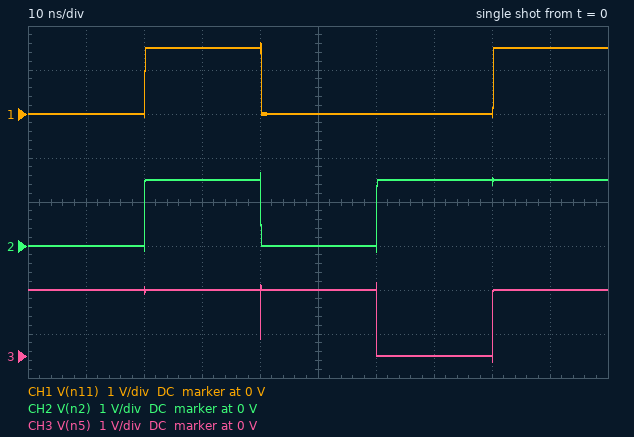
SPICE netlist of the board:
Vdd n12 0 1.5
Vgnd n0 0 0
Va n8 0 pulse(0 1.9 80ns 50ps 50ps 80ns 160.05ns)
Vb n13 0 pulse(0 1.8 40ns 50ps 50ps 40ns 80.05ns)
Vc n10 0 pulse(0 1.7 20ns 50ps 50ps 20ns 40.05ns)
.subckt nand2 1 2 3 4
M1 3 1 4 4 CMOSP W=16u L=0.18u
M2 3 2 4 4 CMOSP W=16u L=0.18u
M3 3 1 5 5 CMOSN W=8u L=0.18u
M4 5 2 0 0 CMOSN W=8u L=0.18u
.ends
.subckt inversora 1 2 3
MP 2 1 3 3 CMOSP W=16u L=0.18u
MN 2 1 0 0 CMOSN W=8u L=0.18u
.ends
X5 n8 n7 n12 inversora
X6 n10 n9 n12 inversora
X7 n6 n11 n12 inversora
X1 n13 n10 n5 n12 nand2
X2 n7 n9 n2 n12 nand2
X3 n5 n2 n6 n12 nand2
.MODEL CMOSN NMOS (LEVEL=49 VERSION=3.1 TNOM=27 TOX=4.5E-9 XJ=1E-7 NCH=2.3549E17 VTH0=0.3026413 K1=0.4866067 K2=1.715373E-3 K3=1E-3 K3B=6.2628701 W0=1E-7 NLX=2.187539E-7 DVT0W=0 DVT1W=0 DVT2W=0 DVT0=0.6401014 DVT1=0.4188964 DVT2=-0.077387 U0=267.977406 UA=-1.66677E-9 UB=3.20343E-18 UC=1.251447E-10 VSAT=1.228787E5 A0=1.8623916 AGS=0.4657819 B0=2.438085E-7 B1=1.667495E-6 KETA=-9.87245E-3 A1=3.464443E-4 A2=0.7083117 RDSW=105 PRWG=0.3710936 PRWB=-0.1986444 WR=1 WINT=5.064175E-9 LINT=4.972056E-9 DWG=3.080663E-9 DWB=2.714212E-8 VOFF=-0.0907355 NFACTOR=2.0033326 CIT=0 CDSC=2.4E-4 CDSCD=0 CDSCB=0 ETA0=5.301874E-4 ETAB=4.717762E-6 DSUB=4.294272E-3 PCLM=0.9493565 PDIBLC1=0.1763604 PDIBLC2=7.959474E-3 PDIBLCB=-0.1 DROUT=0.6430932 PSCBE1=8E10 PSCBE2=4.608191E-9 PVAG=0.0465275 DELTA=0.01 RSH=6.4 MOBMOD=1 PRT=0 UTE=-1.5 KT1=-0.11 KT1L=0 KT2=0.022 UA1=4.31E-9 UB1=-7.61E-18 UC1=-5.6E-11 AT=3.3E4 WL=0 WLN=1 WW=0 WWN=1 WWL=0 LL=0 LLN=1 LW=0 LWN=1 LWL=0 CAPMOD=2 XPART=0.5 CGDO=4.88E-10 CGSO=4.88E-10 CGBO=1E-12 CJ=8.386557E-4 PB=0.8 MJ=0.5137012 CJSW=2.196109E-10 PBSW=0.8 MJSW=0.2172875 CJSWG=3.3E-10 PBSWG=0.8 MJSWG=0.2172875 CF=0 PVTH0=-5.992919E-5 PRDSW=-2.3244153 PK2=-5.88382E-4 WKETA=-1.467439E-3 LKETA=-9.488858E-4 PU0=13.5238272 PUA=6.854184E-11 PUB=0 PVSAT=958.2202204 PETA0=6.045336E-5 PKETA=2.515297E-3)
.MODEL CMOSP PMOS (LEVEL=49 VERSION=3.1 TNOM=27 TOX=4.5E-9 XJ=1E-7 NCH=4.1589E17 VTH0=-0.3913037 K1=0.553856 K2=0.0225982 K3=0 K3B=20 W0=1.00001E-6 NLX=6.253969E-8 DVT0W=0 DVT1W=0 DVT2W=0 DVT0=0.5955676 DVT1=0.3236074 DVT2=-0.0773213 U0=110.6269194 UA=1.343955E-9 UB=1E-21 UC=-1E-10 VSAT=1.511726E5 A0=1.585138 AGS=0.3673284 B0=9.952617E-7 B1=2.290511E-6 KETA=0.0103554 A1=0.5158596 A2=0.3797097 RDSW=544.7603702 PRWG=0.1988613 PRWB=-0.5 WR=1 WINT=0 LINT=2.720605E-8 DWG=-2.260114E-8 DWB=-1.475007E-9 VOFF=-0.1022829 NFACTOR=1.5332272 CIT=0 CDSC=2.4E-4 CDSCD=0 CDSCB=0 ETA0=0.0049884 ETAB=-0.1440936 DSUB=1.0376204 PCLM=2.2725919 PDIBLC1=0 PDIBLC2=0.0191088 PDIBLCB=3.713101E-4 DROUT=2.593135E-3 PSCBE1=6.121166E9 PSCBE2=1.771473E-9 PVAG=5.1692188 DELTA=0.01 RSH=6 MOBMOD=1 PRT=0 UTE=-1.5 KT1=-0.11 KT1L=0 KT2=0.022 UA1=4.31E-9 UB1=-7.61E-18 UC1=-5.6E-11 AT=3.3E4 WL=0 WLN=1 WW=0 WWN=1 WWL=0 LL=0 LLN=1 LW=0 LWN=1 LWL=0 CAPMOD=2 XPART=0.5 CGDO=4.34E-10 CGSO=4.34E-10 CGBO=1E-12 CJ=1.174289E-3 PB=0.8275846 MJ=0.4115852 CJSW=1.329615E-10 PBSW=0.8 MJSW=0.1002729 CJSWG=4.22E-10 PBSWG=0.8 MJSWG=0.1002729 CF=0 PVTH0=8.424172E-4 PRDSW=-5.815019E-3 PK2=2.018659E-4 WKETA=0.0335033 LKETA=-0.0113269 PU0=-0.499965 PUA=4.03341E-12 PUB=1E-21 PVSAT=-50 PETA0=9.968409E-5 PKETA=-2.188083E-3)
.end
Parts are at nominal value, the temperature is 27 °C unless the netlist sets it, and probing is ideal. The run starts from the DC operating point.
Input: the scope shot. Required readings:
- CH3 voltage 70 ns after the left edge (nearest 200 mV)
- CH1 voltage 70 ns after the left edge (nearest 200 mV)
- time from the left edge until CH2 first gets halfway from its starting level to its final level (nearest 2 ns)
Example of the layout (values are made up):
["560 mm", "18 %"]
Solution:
["0 V", "0 V", "20 ns"]
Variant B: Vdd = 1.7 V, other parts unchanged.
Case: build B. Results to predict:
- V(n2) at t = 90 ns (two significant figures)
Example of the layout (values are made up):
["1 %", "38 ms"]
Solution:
["1.7 V"]
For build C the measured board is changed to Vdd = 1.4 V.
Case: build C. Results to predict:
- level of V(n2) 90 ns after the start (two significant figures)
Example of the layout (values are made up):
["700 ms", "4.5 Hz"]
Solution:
["1.4 V"]
